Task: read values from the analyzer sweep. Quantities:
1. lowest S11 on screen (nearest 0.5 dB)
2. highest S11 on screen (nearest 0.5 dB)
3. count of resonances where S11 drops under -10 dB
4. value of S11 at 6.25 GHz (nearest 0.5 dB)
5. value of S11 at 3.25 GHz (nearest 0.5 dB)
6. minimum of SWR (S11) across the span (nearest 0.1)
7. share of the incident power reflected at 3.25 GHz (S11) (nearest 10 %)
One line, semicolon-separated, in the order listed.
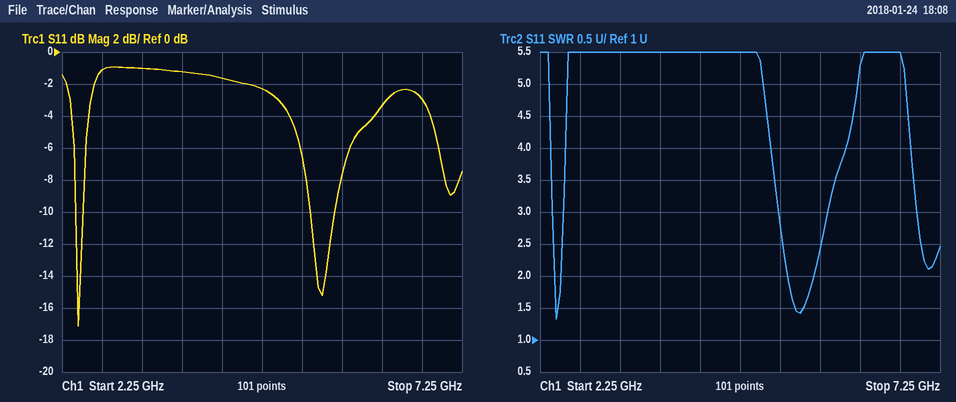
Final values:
-17.0 dB; -1.0 dB; 2; -3.5 dB; -1.0 dB; 1.3; 80 %
